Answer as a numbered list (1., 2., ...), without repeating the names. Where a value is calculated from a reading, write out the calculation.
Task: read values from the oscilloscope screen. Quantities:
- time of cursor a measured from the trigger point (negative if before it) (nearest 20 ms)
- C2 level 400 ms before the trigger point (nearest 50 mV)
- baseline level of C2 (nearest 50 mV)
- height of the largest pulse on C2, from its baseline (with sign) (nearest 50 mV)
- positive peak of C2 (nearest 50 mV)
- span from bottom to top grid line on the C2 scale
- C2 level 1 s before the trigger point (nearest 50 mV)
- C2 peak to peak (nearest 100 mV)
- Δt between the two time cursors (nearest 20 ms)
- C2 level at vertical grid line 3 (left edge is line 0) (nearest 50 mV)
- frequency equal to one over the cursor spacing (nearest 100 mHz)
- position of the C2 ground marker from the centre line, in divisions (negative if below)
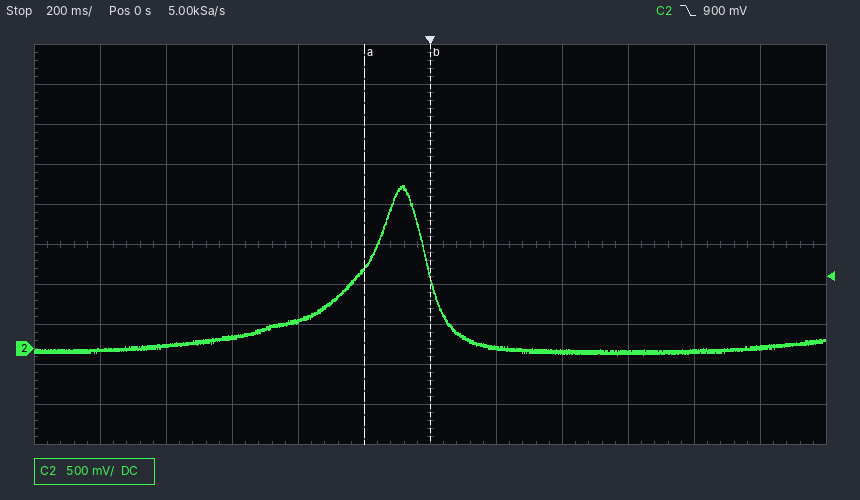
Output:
1. -200 ms
2. 350 mV
3. 0 mV
4. 2.05 V − (0 mV) = +2.05 V
5. 2.05 V
6. 5 V
7. 0 mV
8. 2.10 V
9. 200 ms
10. 150 mV
11. 1 / 200 ms ≈ 5.0 Hz
12. -2.6 div
